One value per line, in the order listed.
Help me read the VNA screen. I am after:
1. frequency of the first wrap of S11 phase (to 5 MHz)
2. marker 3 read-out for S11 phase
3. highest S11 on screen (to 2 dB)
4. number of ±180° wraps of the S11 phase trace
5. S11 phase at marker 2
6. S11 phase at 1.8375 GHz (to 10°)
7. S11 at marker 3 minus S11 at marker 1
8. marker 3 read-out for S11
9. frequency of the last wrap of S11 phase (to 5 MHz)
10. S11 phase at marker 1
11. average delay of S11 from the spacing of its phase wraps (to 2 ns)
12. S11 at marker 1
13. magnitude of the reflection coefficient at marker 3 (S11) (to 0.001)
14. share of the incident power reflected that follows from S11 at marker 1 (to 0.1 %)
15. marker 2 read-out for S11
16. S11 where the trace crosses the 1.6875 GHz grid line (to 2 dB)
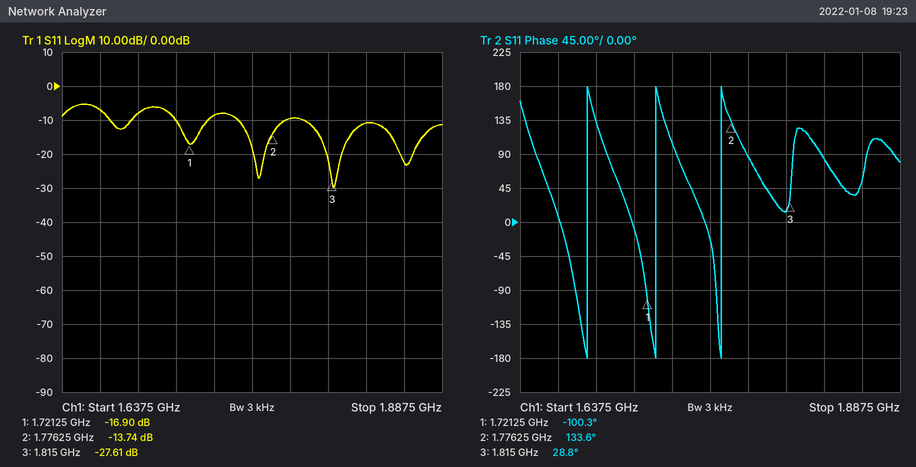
1.680 GHz
28.8°
-6 dB
3
133.6°
80°
-10.71 dB
-27.61 dB
1.770 GHz
-100.3°
22 ns
-16.90 dB
0.042
2.0 %
-13.74 dB
-8 dB
